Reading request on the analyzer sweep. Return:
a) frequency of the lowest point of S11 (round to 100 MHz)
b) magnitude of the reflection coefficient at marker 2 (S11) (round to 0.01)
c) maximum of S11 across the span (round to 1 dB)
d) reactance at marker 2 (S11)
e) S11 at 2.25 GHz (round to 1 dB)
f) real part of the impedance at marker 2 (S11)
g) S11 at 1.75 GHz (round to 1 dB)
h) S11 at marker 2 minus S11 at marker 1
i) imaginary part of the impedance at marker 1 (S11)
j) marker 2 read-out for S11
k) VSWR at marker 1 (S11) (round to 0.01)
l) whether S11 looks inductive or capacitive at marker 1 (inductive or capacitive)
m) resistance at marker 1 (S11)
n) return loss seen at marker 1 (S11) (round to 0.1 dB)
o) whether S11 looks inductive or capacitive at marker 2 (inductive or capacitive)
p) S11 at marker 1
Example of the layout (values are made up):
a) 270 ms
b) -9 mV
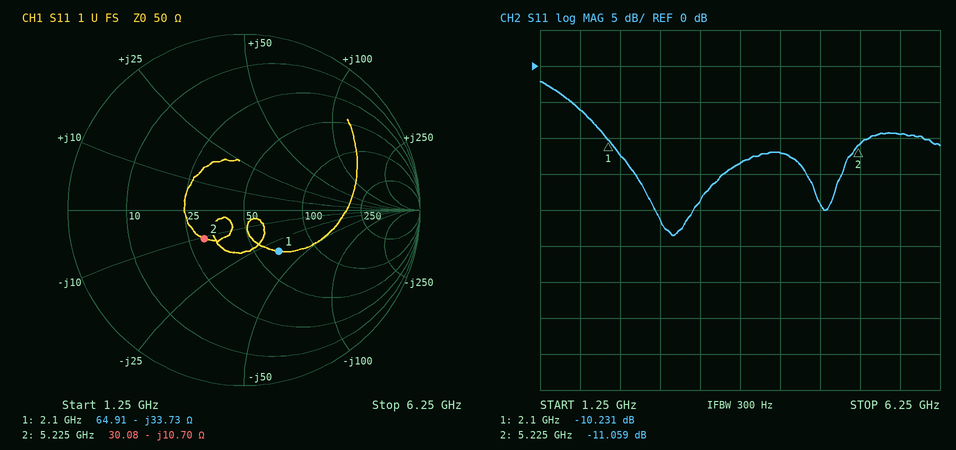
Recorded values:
a) 2.9 GHz
b) 0.28
c) -2 dB
d) -10.70 Ω
e) -12 dB
f) 30.08 Ω
g) -6 dB
h) -0.828 dB
i) -33.73 Ω
j) -11.059 dB
k) 1.89
l) capacitive
m) 64.91 Ω
n) 10.2 dB
o) capacitive
p) -10.231 dB
